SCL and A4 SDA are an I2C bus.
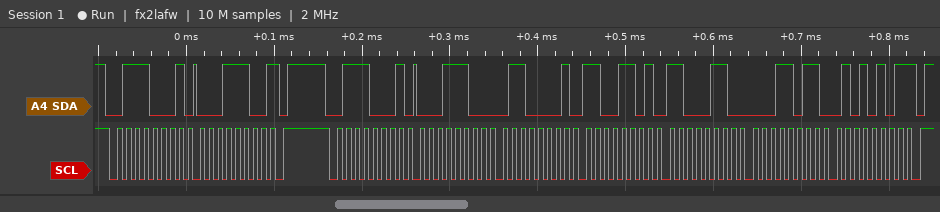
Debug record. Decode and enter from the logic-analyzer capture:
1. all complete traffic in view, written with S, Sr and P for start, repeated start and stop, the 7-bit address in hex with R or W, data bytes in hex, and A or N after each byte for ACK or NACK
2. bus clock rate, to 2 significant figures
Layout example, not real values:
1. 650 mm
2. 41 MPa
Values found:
1. S 38R A 1C N P S 38R A 1C A 61 A CD A C6 A 1B A 55 N P
2. 100 kHz
